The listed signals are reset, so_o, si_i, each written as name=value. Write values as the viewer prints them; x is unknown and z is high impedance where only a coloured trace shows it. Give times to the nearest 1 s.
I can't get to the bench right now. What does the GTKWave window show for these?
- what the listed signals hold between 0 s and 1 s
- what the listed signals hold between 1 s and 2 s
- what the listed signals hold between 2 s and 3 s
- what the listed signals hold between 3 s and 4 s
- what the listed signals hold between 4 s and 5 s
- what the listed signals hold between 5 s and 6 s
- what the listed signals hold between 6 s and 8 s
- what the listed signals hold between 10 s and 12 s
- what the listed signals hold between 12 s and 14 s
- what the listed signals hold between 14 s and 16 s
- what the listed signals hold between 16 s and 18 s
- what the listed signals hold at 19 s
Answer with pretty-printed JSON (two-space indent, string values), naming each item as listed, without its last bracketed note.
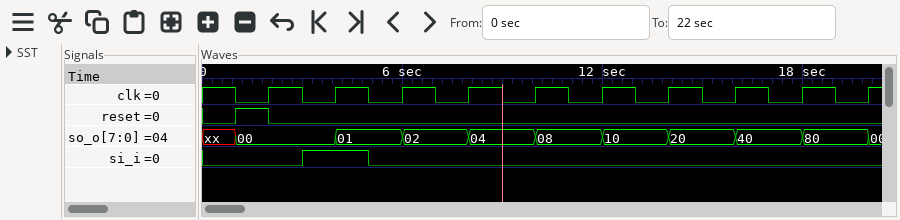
{
  "what the listed signals hold between 0 s and 1 s": "reset=0, so_o=xx, si_i=0",
  "what the listed signals hold between 1 s and 2 s": "reset=1, so_o=00, si_i=0",
  "what the listed signals hold between 2 s and 3 s": "reset=0, so_o=00, si_i=0",
  "what the listed signals hold between 3 s and 4 s": "reset=0, so_o=00, si_i=1",
  "what the listed signals hold between 4 s and 5 s": "reset=0, so_o=01, si_i=1",
  "what the listed signals hold between 5 s and 6 s": "reset=0, so_o=01, si_i=0",
  "what the listed signals hold between 6 s and 8 s": "reset=0, so_o=02, si_i=0",
  "what the listed signals hold between 10 s and 12 s": "reset=0, so_o=08, si_i=0",
  "what the listed signals hold between 12 s and 14 s": "reset=0, so_o=10, si_i=0",
  "what the listed signals hold between 14 s and 16 s": "reset=0, so_o=20, si_i=0",
  "what the listed signals hold between 16 s and 18 s": "reset=0, so_o=40, si_i=0",
  "what the listed signals hold at 19 s": "reset=0, so_o=80, si_i=0"
}
